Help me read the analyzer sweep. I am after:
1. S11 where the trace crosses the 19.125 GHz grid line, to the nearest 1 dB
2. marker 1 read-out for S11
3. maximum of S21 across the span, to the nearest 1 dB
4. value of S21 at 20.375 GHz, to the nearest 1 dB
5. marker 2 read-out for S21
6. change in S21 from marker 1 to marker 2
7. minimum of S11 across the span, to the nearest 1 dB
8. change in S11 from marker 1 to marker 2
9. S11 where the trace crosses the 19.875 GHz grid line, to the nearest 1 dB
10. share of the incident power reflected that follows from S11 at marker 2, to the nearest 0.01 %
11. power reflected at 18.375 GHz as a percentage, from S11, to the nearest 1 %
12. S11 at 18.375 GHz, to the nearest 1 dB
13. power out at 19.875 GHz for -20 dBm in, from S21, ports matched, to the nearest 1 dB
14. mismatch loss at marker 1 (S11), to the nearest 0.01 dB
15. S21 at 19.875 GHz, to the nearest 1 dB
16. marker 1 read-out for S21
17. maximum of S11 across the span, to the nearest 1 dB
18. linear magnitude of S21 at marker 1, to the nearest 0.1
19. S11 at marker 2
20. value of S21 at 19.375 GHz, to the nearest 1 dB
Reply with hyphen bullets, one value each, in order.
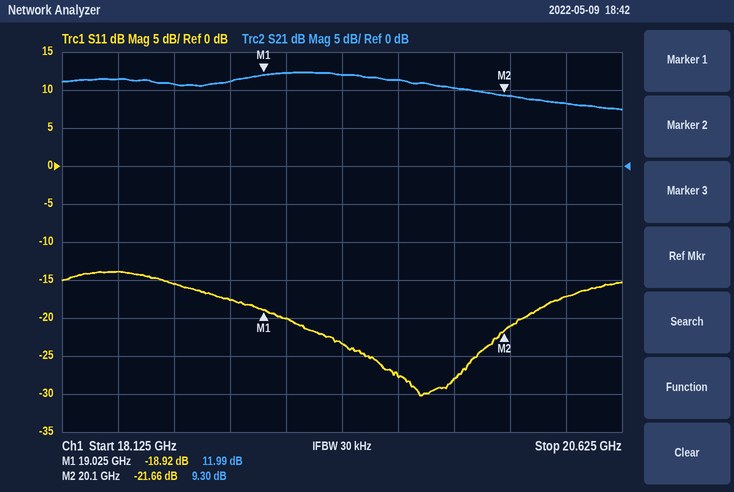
- -20 dB
- -18.92 dB
- 12 dB
- 8 dB
- 9.30 dB
- -2.69 dB
- -30 dB
- -2.74 dB
- -28 dB
- 0.68 %
- 4 %
- -14 dB
- -10 dBm
- 0.06 dB
- 10 dB
- 11.99 dB
- -14 dB
- 4.0
- -21.66 dB
- 12 dB
